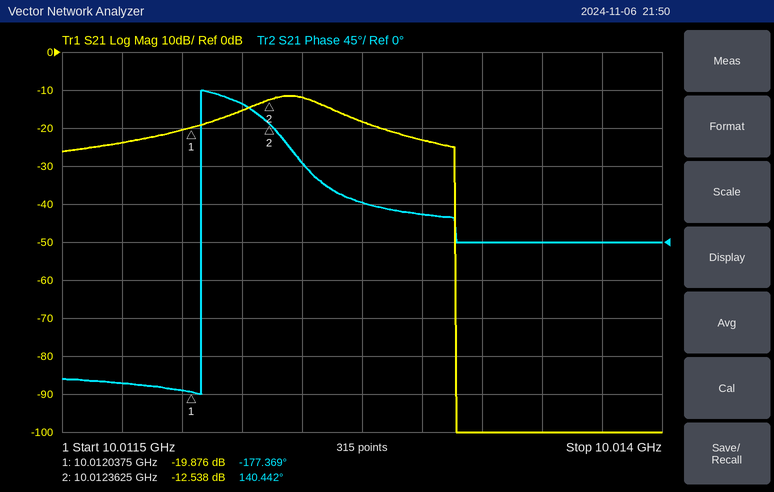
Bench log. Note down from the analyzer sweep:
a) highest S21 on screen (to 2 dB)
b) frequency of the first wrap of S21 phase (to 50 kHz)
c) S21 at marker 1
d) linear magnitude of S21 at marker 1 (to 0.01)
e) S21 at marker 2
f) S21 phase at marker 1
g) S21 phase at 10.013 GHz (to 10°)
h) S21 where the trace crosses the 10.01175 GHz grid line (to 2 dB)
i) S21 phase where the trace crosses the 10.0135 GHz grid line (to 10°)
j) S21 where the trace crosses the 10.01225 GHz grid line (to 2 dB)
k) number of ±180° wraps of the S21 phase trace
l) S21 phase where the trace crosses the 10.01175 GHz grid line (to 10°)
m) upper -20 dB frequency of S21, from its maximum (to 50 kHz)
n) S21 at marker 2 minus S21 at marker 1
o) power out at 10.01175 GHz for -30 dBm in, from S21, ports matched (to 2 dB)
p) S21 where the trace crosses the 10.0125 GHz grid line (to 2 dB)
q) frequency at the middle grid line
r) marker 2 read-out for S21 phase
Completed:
-12 dB
10.01210 GHz
-19.876 dB
0.10
-12.538 dB
-177.369°
30°
-24 dB
0°
-16 dB
1
-170°
10.01315 GHz
7.338 dB
-54 dBm
-12 dB
10.01275 GHz
140.442°
